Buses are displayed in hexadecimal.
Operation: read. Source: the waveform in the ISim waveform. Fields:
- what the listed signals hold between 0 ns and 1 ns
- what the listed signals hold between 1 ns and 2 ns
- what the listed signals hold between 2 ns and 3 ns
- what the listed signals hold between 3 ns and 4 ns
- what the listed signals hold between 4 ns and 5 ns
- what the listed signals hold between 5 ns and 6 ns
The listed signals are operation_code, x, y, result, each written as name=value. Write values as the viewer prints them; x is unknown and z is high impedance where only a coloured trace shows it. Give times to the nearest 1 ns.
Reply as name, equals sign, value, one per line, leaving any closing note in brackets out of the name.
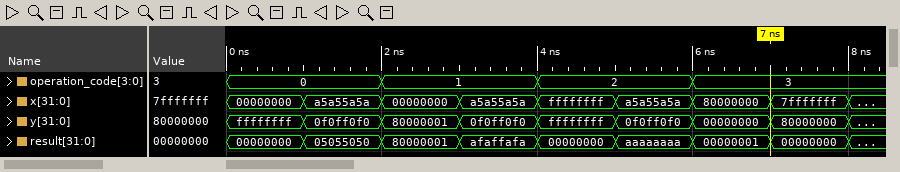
what the listed signals hold between 0 ns and 1 ns = operation_code=0, x=00000000, y=ffffffff, result=00000000
what the listed signals hold between 1 ns and 2 ns = operation_code=0, x=a5a55a5a, y=0f0ff0f0, result=05055050
what the listed signals hold between 2 ns and 3 ns = operation_code=1, x=00000000, y=80000001, result=80000001
what the listed signals hold between 3 ns and 4 ns = operation_code=1, x=a5a55a5a, y=0f0ff0f0, result=afaffafa
what the listed signals hold between 4 ns and 5 ns = operation_code=2, x=ffffffff, y=ffffffff, result=00000000
what the listed signals hold between 5 ns and 6 ns = operation_code=2, x=a5a55a5a, y=0f0ff0f0, result=aaaaaaaa
